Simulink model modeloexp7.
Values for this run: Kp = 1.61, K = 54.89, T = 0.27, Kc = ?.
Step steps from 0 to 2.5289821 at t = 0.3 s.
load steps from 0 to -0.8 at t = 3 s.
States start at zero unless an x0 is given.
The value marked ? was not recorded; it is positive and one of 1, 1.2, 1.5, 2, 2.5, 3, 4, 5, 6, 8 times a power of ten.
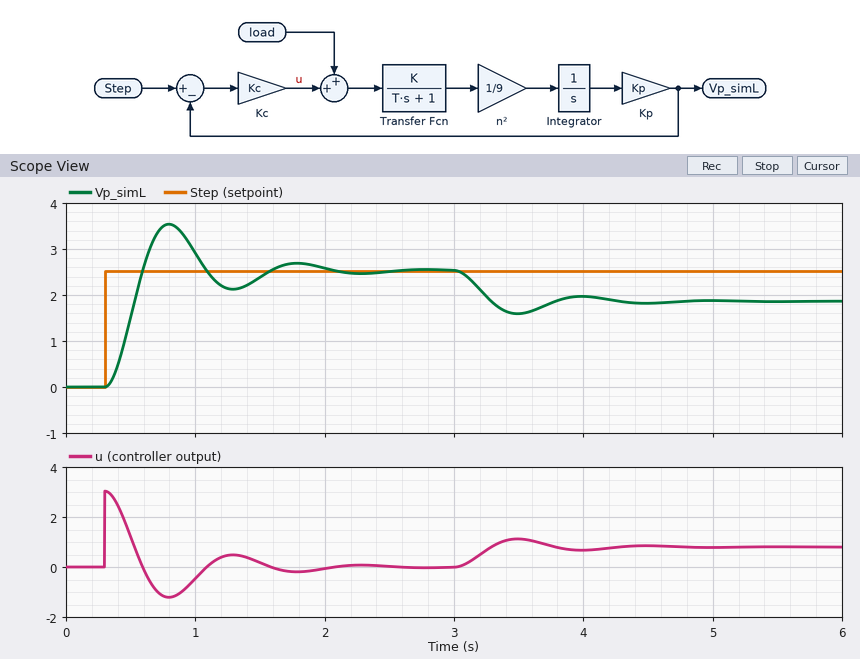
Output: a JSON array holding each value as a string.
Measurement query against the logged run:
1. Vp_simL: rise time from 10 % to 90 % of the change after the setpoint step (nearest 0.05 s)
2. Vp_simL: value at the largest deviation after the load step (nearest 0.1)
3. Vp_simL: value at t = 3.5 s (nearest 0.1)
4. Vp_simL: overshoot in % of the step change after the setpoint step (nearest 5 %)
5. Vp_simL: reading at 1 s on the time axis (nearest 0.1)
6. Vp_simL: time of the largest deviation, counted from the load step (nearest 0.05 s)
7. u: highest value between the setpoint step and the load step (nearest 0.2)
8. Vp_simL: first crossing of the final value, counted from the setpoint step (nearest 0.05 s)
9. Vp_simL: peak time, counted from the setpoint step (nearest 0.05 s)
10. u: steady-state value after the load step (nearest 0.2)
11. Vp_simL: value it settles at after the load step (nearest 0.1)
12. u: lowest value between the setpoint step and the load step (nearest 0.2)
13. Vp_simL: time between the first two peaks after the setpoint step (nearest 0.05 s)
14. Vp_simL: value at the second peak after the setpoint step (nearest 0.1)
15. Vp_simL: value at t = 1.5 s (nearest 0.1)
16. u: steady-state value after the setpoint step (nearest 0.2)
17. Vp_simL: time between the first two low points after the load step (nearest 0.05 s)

["0.20 s", "1.6", "1.6", "40 %", "2.9", "0.50 s", "3.0", "0.30 s", "0.50 s", "0.8", "1.9", "-1.2", "1.00 s", "2.7", "2.4", "0.0", "1.00 s"]
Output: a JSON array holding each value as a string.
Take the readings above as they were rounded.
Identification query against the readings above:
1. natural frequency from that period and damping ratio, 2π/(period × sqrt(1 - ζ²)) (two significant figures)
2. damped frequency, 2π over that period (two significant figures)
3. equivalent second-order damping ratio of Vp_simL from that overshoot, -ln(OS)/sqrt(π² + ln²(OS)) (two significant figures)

["6.5 rad/s", "6.3 rad/s", "0.28"]
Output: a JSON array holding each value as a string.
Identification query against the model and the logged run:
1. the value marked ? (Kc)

["1.2"]
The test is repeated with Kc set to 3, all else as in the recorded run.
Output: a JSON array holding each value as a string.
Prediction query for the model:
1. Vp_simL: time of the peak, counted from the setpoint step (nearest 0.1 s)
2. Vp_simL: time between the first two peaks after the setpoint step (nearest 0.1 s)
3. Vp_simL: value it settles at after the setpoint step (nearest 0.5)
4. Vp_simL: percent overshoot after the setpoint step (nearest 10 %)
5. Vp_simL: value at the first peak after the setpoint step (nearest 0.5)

["0.3 s", "0.6 s", "2.5", "60 %", "4.0"]
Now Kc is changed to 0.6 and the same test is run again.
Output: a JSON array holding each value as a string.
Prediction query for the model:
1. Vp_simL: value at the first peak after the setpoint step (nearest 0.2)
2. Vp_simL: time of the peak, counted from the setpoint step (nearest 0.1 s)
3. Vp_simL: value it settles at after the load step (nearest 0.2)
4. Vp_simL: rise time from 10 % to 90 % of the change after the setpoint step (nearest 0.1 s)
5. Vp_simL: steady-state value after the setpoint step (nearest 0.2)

["3.2", "0.7 s", "1.2", "0.3 s", "2.6"]
